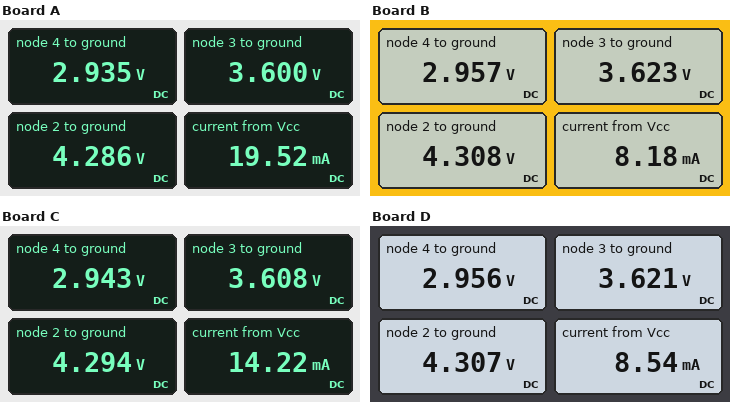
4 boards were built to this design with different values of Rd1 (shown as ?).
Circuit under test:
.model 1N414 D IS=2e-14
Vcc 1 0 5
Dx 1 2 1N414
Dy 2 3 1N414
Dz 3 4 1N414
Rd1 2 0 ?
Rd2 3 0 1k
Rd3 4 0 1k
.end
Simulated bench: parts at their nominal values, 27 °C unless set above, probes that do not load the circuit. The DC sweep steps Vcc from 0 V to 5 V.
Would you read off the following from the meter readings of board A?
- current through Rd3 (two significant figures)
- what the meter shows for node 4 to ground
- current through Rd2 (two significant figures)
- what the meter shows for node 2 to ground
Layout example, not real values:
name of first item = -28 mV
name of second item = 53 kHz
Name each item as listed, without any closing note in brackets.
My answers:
current through Rd3 = 2.9 mA
what the meter shows for node 4 to ground = 2.935 V
current through Rd2 = 3.6 mA
what the meter shows for node 2 to ground = 4.286 V
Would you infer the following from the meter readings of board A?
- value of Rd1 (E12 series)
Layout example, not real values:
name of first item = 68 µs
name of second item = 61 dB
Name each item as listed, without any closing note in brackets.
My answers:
value of Rd1 = 330 Ω
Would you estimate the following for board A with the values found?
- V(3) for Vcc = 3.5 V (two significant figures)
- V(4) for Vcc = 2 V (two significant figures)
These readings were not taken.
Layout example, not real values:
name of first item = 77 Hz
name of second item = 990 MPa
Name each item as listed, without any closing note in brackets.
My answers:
V(3) for Vcc = 3.5 V = 2.1 V
V(4) for Vcc = 2 V = 110 mV
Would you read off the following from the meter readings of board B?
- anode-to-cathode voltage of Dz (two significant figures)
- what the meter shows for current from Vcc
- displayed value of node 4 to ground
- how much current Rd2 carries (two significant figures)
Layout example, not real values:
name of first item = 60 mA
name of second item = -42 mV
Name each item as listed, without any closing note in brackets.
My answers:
anode-to-cathode voltage of Dz = 670 mV
what the meter shows for current from Vcc = 8.18 mA
displayed value of node 4 to ground = 2.957 V
how much current Rd2 carries = 3.6 mA
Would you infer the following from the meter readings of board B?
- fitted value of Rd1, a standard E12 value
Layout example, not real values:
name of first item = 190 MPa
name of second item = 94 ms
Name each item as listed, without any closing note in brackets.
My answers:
fitted value of Rd1, a standard E12 value = 2.7 kΩ
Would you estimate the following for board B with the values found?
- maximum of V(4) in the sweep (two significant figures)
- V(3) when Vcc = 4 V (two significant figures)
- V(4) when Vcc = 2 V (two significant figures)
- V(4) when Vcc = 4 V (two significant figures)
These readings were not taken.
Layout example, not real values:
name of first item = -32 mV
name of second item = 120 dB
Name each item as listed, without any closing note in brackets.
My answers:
maximum of V(4) in the sweep = 3.0 V
V(3) when Vcc = 4 V = 2.6 V
V(4) when Vcc = 2 V = 140 mV
V(4) when Vcc = 4 V = 2.0 V
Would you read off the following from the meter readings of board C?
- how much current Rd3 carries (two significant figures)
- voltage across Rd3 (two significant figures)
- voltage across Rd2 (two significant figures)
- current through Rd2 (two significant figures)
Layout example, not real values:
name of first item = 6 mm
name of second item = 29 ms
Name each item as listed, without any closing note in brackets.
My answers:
how much current Rd3 carries = 2.9 mA
voltage across Rd3 = 2.9 V
voltage across Rd2 = 3.6 V
current through Rd2 = 3.6 mA
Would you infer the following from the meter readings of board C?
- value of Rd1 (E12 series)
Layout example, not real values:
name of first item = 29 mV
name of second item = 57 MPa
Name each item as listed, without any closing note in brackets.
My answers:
value of Rd1 = 560 Ω
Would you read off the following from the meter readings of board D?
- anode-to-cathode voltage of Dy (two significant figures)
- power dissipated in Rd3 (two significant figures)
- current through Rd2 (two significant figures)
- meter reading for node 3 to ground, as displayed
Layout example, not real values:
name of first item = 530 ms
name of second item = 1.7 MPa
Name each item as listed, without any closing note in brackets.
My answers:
anode-to-cathode voltage of Dy = 690 mV
power dissipated in Rd3 = 8.7 mW
current through Rd2 = 3.6 mA
meter reading for node 3 to ground, as displayed = 3.621 V
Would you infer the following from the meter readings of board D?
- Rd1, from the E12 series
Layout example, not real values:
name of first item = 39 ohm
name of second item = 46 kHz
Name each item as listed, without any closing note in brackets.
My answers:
Rd1, from the E12 series = 2.2 kΩ
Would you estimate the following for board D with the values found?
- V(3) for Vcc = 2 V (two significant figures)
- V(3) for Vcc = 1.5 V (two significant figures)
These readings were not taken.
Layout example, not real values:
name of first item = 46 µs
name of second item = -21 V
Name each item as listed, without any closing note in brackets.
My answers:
V(3) for Vcc = 2 V = 720 mV
V(3) for Vcc = 1.5 V = 270 mV
